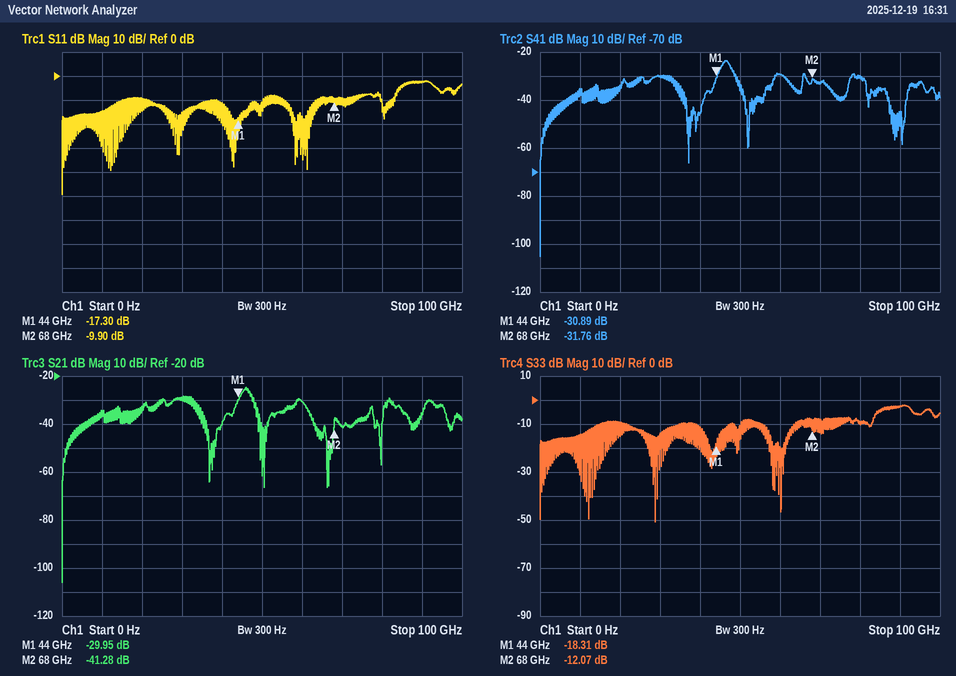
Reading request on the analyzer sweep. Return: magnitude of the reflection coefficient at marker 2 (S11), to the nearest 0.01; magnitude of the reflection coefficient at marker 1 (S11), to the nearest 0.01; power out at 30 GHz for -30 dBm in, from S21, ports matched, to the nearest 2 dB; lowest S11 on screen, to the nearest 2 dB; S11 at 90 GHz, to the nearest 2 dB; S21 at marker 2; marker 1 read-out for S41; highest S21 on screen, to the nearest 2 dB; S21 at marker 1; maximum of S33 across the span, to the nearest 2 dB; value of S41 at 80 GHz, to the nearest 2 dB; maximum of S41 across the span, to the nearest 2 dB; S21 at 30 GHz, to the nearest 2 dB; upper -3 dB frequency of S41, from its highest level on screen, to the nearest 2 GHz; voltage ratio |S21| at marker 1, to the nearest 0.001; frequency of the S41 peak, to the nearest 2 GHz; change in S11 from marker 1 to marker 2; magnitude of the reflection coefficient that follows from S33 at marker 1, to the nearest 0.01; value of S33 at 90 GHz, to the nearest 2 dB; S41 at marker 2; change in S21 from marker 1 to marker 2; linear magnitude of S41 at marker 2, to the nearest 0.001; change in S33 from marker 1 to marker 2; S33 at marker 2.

0.32
0.14
-60 dBm
-50 dB
-2 dB
-41.28 dB
-30.89 dB
-24 dB
-29.95 dB
-2 dB
-30 dB
-24 dB
-30 dB
48 GHz
0.032
46 GHz
7.40 dB
0.12
-2 dB
-31.76 dB
-11.33 dB
0.026
6.24 dB
-12.07 dB
